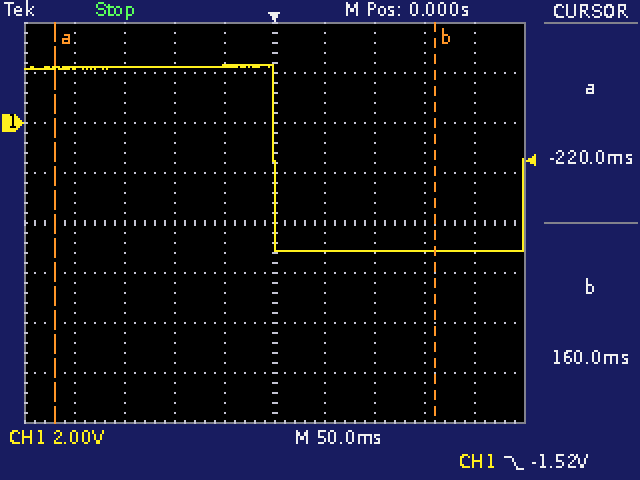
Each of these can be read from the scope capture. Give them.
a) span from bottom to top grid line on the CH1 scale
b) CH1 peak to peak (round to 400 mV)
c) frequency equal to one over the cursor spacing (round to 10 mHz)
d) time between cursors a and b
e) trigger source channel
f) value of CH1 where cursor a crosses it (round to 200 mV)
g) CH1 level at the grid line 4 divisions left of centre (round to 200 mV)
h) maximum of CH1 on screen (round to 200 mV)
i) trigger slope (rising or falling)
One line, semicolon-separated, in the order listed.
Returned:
16 V; 7.6 V; 2.63 Hz; 380 ms; CH1; 2.2 V; 2.2 V; 2.4 V; falling
